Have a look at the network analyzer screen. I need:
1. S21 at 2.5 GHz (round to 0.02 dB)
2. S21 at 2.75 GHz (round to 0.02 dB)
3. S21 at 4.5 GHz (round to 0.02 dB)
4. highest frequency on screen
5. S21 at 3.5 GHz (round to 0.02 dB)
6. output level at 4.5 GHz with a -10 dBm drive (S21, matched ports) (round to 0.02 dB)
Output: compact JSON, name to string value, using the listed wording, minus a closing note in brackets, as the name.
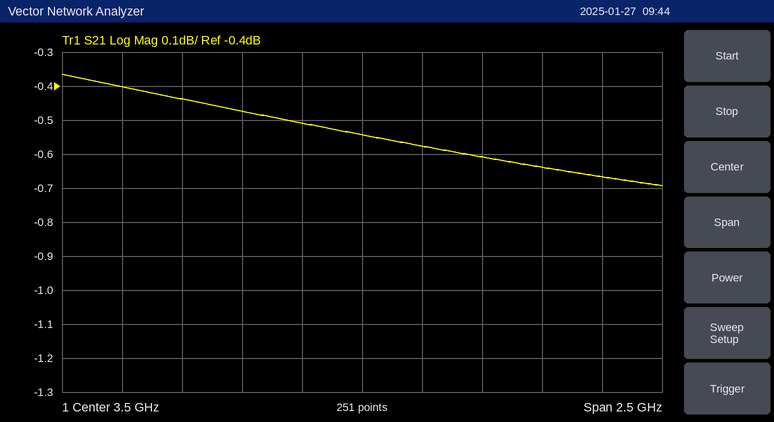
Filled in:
{"S21 at 2.5 GHz": "-0.40 dB", "S21 at 2.75 GHz": "-0.44 dB", "S21 at 4.5 GHz": "-0.66 dB", "highest frequency on screen": "4.75 GHz", "S21 at 3.5 GHz": "-0.54 dB", "output level at 4.5 GHz with a -10 dBm drive (S21, matched ports)": "-10.66 dBm"}
